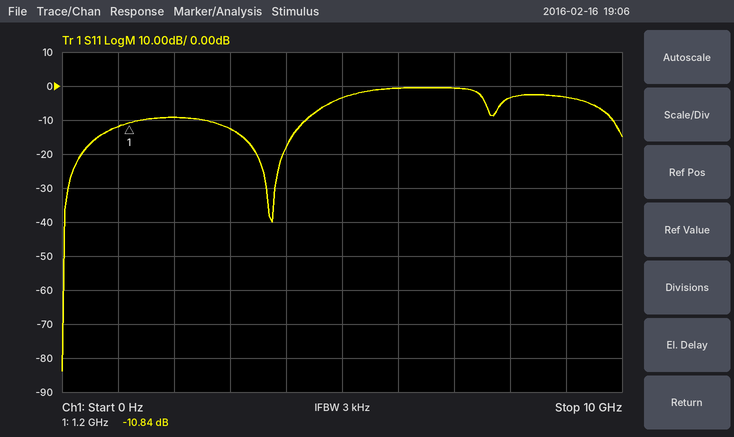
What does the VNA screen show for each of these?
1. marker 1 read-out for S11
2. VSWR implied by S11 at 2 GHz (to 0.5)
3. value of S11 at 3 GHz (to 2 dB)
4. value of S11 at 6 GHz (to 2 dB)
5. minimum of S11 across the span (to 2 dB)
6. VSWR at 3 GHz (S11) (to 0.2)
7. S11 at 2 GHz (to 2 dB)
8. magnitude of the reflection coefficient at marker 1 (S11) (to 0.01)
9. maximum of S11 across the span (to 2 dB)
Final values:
-10.84 dB
2.0
-12 dB
0 dB
-84 dB
1.6
-10 dB
0.29
0 dB
